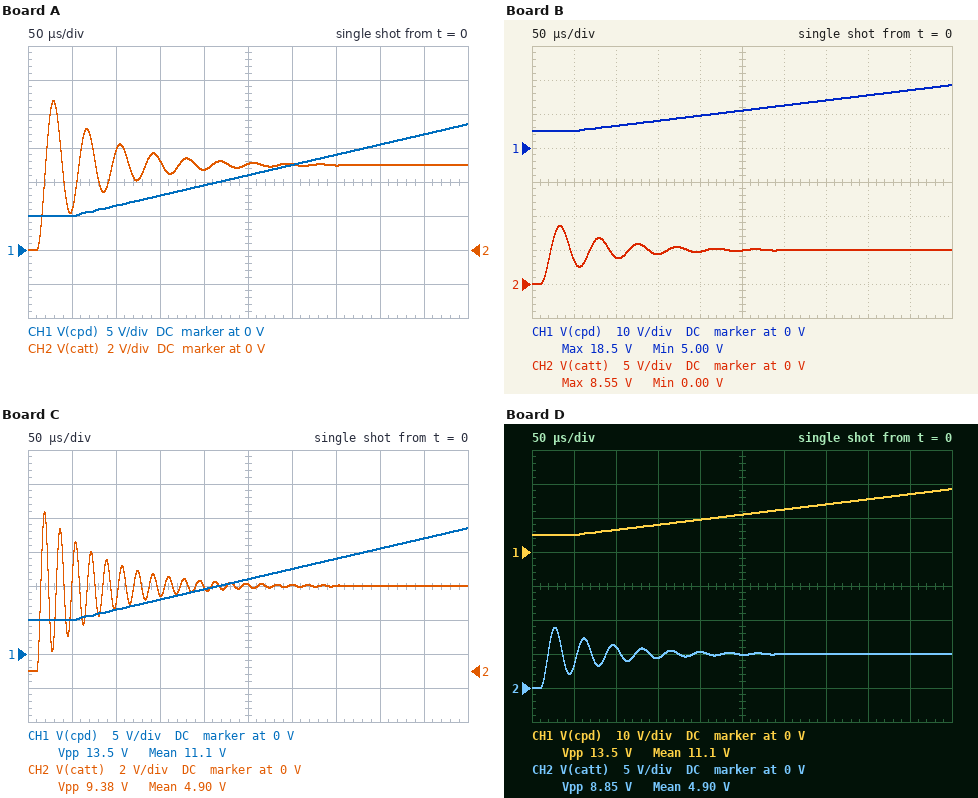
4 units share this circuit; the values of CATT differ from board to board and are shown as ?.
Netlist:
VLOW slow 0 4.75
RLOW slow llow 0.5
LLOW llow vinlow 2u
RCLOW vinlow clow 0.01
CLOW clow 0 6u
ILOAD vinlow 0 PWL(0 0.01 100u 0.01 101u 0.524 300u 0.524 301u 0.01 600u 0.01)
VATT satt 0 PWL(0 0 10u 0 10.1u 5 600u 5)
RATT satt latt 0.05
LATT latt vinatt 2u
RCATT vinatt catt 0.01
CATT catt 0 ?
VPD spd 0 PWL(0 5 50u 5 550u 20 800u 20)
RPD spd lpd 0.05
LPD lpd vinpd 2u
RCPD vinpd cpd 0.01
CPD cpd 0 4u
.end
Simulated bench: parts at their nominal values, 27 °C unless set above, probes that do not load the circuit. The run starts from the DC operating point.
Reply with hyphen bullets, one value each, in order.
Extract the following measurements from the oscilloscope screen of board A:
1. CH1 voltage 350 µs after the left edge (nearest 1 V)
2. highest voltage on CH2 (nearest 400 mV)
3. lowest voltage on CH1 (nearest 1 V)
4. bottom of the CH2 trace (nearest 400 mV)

- 14 V
- 8.8 V
- 5 V
- 0 V
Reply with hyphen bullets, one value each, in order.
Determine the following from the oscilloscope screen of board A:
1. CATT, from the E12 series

- 18 µF
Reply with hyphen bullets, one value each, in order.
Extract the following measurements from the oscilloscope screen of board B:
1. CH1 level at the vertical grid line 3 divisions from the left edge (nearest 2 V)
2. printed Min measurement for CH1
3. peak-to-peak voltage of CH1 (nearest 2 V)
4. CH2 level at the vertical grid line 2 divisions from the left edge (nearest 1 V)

- 8 V
- 5.00 V
- 14 V
- 4 V
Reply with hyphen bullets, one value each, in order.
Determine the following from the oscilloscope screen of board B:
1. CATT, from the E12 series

- 27 µF
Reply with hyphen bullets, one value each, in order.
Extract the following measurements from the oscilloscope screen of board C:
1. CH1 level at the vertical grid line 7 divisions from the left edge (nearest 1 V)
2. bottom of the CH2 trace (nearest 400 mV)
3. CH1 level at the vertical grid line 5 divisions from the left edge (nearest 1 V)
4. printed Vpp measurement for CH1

- 14 V
- 0 V
- 11 V
- 13.5 V
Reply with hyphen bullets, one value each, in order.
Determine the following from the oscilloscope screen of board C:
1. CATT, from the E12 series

- 3.9 µF
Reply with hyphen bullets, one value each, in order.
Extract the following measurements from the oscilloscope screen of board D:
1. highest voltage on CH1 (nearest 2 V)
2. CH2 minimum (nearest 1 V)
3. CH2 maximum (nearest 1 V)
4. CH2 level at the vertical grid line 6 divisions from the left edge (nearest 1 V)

- 18 V
- 0 V
- 9 V
- 5 V
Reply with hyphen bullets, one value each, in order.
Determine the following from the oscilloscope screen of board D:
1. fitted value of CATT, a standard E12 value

- 15 µF
